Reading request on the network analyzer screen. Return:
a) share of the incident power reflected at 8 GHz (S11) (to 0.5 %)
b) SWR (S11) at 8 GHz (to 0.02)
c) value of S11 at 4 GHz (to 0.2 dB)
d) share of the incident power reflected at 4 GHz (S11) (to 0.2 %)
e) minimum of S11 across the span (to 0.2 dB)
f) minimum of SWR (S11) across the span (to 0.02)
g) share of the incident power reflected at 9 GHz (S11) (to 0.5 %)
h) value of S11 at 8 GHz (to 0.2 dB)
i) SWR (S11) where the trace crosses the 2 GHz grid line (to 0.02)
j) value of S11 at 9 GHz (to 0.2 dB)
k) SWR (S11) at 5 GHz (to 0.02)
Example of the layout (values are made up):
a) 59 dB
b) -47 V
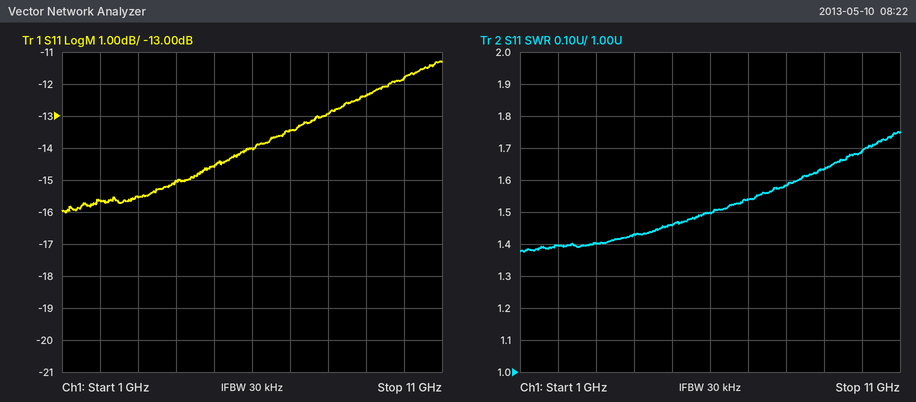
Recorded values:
a) 5.0 %
b) 1.58
c) -15.0 dB
d) 3.2 %
e) -16.0 dB
f) 1.38
g) 6.0 %
h) -13.0 dB
i) 1.40
j) -12.4 dB
k) 1.46
